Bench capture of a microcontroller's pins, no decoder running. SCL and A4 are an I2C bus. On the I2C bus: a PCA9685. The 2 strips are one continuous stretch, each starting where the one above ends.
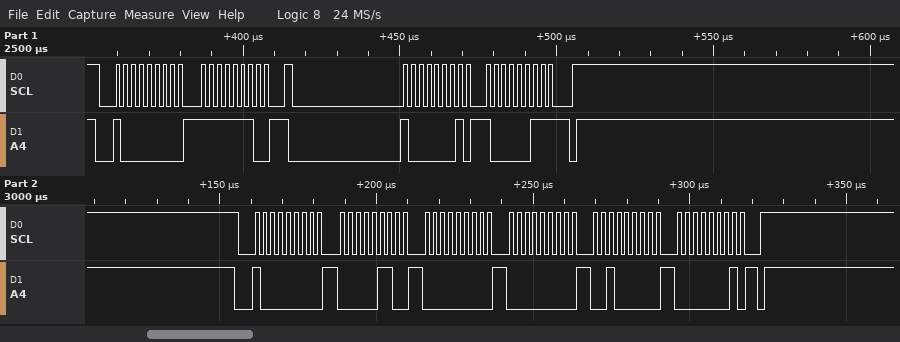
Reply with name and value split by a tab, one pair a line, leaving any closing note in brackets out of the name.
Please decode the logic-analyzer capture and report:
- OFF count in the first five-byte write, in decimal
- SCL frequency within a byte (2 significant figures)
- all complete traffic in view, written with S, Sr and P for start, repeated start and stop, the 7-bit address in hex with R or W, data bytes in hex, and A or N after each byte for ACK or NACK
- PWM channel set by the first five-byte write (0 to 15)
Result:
OFF count in the first five-byte write, in decimal	288
SCL frequency within a byte	400 kHz
all complete traffic in view, written with S, Sr and P for start, repeated start and stop, the 7-bit address in hex with R or W, data bytes in hex, and A or N after each byte for ACK or NACK	S 40W A FE A Sr 40R A 83 N P S 40W A 06 A 00 A 00 A 20 A 01 A P
PWM channel set by the first five-byte write	0
